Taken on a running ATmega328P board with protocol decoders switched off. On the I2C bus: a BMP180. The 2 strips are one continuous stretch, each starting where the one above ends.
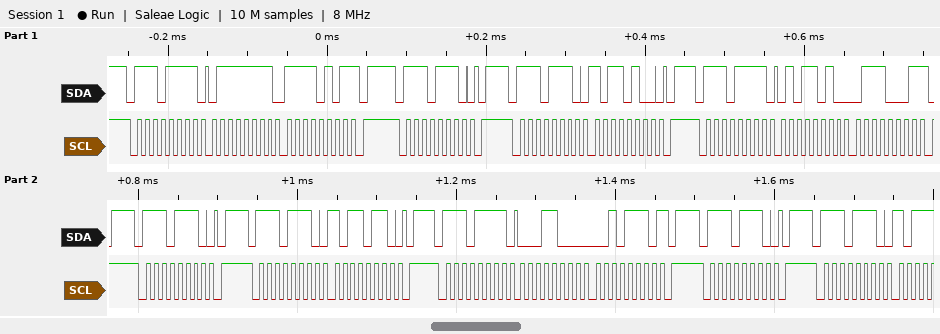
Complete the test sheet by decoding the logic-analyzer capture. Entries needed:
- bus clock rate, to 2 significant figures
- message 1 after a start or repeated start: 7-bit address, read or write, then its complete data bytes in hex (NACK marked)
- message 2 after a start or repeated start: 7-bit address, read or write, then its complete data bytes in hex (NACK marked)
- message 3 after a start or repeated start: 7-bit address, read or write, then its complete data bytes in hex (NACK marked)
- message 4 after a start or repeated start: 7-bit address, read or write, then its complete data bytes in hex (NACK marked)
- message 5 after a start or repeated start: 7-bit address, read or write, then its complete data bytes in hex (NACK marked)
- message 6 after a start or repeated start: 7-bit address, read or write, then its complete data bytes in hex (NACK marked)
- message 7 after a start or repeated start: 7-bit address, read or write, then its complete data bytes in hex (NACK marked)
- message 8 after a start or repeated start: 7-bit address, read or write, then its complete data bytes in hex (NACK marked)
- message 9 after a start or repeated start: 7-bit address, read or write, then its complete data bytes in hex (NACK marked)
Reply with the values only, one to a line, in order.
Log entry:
100 kHz
0x77 read: 7F F5 NACK
0x77 write
0x77 write: B4
0x77 read: 5A 71 NACK
0x77 write
0x77 write: B6
0x77 read: 18 2E NACK
0x77 write
0x77 write
